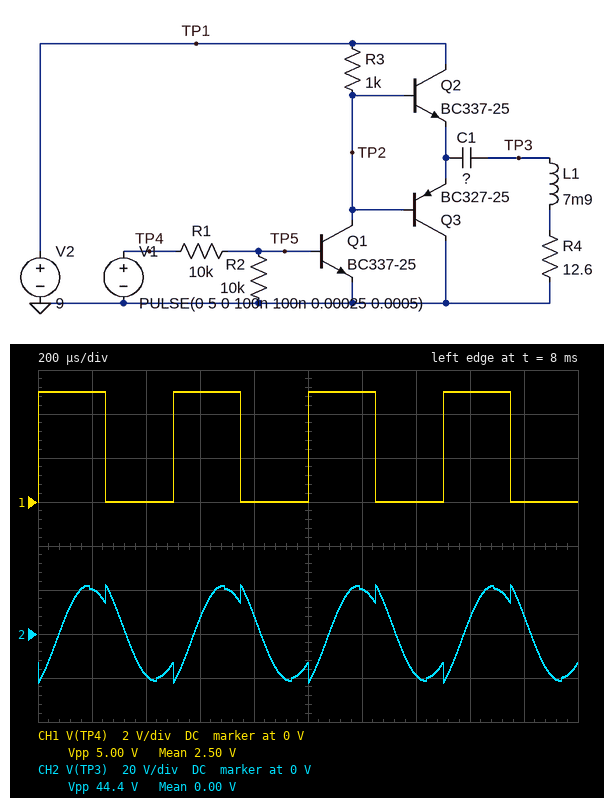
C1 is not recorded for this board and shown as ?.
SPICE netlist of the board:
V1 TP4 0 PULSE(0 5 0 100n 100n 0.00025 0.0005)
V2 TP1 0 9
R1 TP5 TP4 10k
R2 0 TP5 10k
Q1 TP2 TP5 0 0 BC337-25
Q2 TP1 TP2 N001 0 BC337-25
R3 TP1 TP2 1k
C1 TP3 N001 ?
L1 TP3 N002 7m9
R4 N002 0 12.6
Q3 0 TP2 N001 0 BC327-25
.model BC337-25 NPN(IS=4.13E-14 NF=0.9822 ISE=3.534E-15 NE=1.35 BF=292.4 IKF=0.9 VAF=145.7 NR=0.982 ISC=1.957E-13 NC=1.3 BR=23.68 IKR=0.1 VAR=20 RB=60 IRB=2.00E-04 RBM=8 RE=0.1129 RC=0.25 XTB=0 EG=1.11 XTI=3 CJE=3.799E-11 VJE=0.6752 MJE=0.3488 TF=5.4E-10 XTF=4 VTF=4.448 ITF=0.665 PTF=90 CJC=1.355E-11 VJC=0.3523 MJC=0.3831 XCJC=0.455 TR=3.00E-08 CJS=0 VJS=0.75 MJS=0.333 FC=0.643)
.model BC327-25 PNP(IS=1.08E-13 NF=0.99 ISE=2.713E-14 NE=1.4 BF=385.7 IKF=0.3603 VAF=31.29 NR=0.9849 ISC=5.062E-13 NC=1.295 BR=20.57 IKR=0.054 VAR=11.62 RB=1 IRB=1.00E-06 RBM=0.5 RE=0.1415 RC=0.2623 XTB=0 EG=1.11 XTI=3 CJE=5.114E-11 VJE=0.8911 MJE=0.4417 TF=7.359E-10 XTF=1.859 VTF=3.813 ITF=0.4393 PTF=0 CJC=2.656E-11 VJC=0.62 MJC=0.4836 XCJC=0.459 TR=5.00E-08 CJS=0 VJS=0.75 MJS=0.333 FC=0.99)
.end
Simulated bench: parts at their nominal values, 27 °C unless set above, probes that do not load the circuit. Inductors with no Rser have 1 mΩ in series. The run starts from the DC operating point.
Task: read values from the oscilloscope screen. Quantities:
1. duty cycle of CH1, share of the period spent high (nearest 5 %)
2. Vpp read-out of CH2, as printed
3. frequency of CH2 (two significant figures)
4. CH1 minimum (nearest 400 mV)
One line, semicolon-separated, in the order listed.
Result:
50 %; 44.4 V; 2.0 kHz; 0 V
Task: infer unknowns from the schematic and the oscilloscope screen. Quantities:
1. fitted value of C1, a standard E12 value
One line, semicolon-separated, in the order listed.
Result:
680 nF
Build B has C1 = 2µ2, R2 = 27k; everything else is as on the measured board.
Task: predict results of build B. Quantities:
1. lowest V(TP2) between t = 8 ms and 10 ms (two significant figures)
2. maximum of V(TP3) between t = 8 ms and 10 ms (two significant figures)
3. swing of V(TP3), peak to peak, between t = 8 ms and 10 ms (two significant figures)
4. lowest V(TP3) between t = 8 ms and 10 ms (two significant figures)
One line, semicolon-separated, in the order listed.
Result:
26 mV; 8.2 V; 16 V; -8.0 V
